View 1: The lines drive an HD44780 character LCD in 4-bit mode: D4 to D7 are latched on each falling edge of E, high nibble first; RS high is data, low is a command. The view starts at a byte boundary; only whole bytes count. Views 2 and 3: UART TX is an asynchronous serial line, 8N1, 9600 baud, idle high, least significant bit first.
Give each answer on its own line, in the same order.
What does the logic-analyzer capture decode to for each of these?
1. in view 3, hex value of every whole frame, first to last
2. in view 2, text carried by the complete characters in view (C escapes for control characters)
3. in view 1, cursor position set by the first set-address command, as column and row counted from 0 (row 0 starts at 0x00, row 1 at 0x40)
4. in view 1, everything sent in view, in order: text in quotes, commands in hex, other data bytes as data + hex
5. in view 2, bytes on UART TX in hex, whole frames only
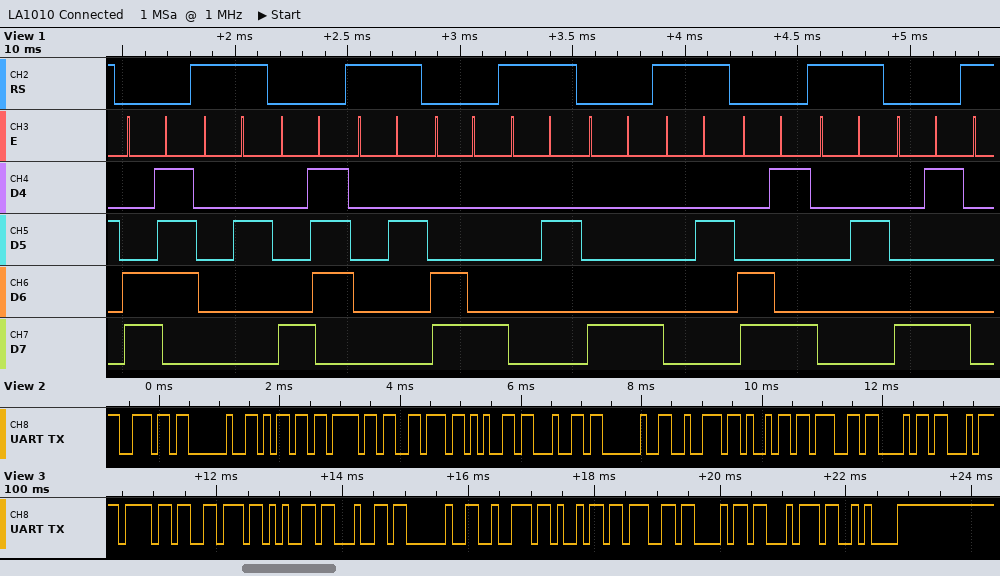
6F 76 65 64 20 72 69 67 68 74 0A
"n moved righ"
column 7, row 1
0xC7 data 02 0x87 data 02 0xC8 data 02 0x88 data 02 0xC9 data 02 0x89
6E 20 6D 6F 76 65 64 20 72 69 67 68
